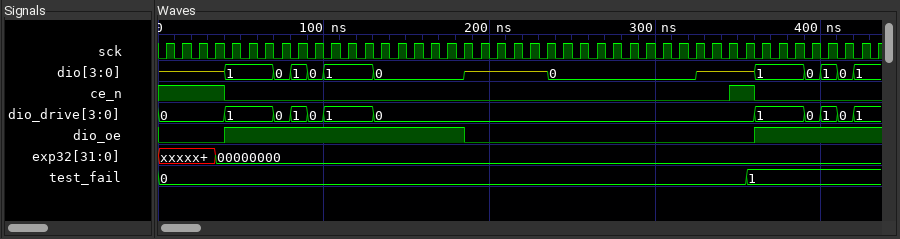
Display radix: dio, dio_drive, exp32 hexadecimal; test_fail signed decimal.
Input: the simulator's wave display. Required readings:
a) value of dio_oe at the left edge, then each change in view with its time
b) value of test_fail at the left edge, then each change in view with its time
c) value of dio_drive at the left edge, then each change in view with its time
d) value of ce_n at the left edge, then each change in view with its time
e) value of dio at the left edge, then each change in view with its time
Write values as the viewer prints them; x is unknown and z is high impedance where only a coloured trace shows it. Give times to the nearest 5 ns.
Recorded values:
0, 1 at 40 ns, 0 at 185 ns, 1 at 360 ns
0, 1 at 355 ns
0, 1 at 40 ns, 0 at 70 ns, 1 at 80 ns, 0 at 90 ns, 1 at 100 ns, 0 at 130 ns, 1 at 360 ns, 0 at 390 ns, 1 at 400 ns, 0 at 410 ns, 1 at 420 ns
1, 0 at 40 ns, 1 at 345 ns, 0 at 360 ns
z, 1 at 40 ns, 0 at 70 ns, 1 at 80 ns, 0 at 90 ns, 1 at 100 ns, 0 at 130 ns, z at 185 ns, 0 at 235 ns, z at 325 ns, 1 at 360 ns, 0 at 390 ns, 1 at 400 ns, 0 at 410 ns, 1 at 420 ns
